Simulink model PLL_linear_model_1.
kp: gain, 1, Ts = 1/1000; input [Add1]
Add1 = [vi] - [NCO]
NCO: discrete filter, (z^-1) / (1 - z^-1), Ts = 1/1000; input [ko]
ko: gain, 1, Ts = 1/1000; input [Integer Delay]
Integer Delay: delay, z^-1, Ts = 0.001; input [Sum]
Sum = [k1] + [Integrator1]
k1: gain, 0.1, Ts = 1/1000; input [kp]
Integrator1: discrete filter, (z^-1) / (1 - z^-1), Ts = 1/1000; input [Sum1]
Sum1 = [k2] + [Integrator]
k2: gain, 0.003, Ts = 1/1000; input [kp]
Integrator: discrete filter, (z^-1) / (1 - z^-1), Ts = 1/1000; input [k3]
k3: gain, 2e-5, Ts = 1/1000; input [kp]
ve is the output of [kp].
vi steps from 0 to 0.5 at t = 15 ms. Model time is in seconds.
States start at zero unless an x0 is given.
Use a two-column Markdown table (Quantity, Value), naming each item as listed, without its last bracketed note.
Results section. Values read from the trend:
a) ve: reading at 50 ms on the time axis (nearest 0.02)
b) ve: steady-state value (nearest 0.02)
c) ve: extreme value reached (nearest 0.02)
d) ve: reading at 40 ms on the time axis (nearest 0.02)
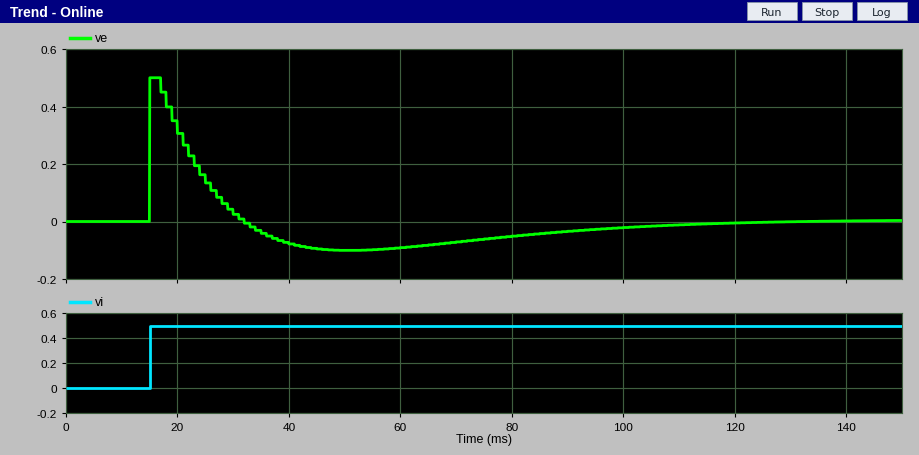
| Quantity | Value |
|---|---|
| ve: reading at 50 ms on the time axis | -0.10 |
| ve: steady-state value | 0.00 |
| ve: extreme value reached | 0.50 |
| ve: reading at 40 ms on the time axis | -0.08 |
